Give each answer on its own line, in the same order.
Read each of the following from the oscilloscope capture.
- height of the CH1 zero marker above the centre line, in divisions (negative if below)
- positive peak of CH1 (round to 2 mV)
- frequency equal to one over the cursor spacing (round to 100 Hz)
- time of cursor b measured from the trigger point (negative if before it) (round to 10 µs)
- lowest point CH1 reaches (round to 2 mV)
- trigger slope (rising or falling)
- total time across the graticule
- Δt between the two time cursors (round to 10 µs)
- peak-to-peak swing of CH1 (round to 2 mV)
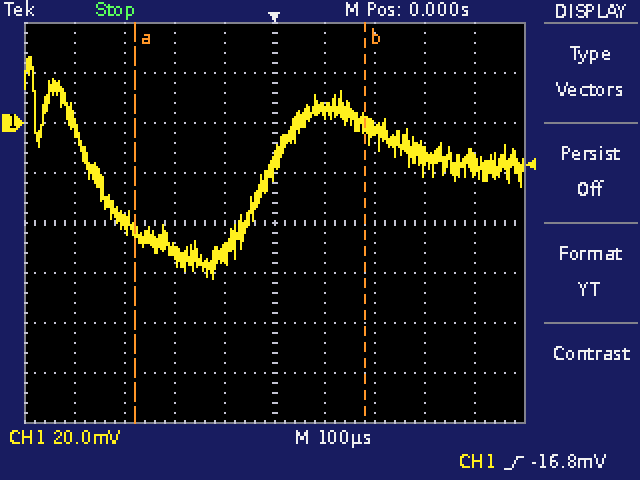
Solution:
+2.0 div
26 mV
2.2 kHz
+180 µs
-62 mV
rising
1 ms
460 µs
88 mV
